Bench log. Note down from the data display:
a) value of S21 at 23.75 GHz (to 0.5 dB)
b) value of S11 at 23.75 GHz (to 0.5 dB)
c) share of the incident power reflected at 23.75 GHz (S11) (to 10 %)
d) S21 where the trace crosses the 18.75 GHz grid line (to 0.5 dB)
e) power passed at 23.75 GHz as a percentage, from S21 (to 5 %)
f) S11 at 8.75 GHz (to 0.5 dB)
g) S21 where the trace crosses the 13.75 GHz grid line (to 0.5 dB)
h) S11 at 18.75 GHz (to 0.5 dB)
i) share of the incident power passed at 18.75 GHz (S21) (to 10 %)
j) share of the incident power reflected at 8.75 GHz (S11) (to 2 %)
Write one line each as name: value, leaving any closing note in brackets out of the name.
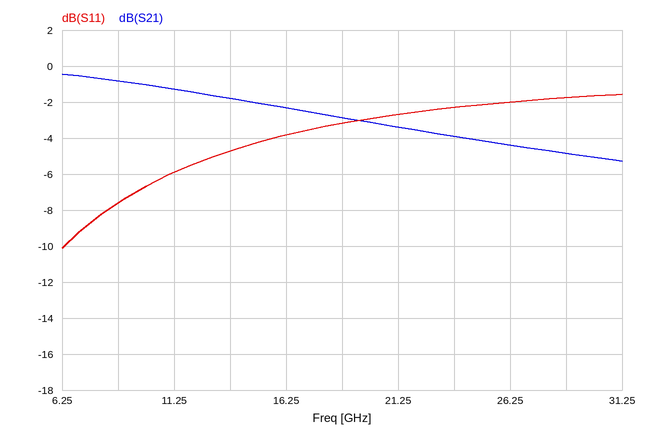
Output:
value of S21 at 23.75 GHz: -4.0 dB
value of S11 at 23.75 GHz: -2.5 dB
share of the incident power reflected at 23.75 GHz (S11): 60 %
S21 where the trace crosses the 18.75 GHz grid line: -3.0 dB
power passed at 23.75 GHz as a percentage, from S21: 40 %
S11 at 8.75 GHz: -7.5 dB
S21 where the trace crosses the 13.75 GHz grid line: -2.0 dB
S11 at 18.75 GHz: -3.0 dB
share of the incident power passed at 18.75 GHz (S21): 50 %
share of the incident power reflected at 8.75 GHz (S11): 18 %
